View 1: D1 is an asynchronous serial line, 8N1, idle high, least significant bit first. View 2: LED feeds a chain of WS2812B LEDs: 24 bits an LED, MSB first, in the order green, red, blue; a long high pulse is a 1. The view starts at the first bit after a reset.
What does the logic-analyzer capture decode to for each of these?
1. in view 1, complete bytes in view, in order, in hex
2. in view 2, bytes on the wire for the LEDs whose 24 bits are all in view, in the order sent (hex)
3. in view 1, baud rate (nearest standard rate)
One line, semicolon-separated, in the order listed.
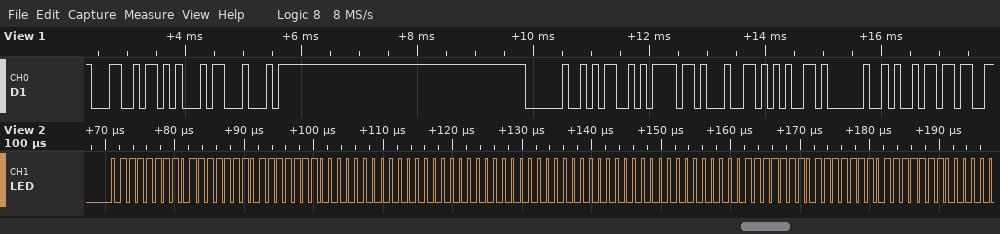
4C 45 44 20 4D 6F 64 65 20 69; 7F 7F 7F 00 00 00 00 00 00 7F 7F 7F; 9600 baud
